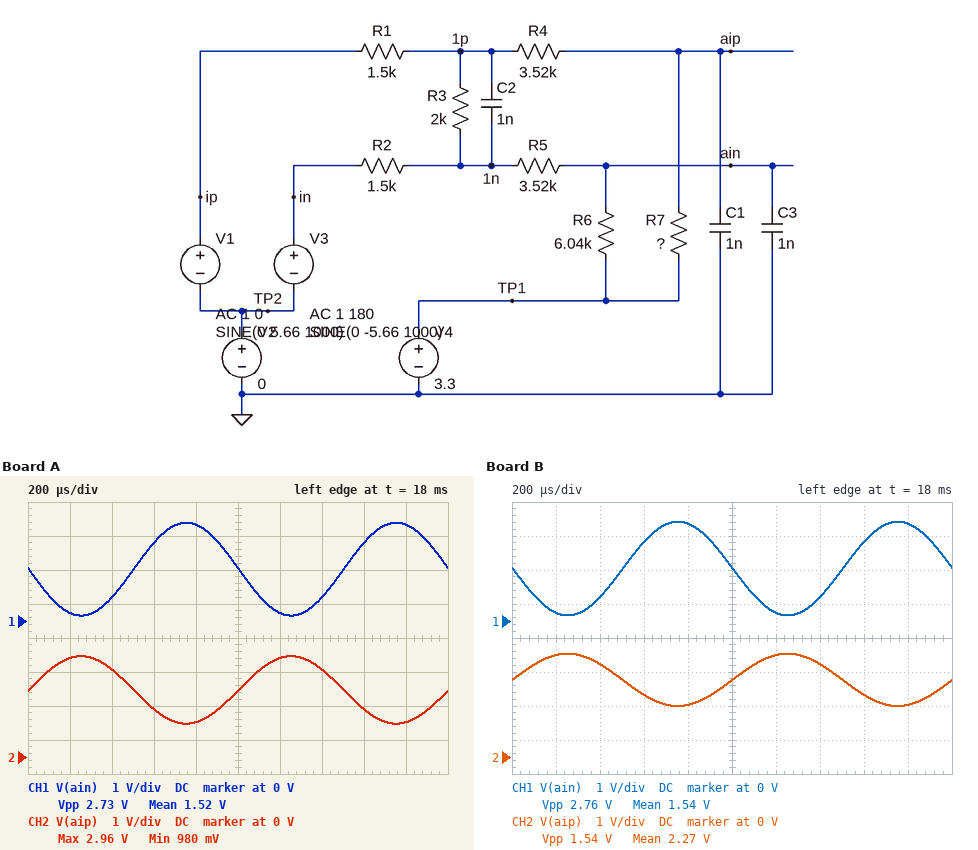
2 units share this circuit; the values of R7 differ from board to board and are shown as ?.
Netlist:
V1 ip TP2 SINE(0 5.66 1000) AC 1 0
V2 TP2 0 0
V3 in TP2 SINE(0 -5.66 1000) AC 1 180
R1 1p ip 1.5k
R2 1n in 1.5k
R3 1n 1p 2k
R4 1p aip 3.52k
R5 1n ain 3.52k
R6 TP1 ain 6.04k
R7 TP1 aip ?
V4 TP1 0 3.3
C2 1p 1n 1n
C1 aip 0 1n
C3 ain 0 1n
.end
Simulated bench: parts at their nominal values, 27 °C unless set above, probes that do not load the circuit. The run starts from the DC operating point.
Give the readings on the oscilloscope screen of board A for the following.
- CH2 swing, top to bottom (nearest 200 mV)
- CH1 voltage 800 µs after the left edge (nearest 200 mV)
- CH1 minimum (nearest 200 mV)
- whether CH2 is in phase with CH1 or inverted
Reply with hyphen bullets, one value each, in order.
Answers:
- 2.0 V
- 2.8 V
- 200 mV
- inverted
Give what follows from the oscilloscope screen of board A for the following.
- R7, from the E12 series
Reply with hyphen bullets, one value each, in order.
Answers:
- 3.3 kΩ
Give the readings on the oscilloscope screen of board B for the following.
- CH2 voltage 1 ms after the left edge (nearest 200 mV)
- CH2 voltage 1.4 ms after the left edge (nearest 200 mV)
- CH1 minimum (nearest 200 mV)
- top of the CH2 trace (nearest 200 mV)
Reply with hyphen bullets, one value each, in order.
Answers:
- 2.2 V
- 2.8 V
- 200 mV
- 3.0 V
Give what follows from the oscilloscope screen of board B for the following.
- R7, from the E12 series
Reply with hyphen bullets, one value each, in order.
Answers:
- 2.2 kΩ
